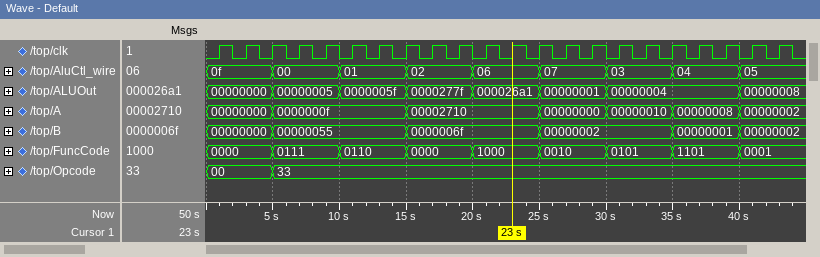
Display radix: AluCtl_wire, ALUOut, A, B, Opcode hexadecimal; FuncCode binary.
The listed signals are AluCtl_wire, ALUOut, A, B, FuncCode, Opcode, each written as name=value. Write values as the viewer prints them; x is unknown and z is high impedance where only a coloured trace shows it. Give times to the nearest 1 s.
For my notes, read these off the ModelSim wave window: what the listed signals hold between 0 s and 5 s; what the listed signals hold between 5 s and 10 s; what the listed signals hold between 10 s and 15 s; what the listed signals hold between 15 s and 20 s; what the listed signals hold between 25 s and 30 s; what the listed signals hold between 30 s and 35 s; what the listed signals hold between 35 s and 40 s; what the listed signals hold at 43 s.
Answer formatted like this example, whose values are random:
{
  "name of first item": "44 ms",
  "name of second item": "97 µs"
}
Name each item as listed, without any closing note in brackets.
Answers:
{
  "what the listed signals hold between 0 s and 5 s": "AluCtl_wire=0f, ALUOut=00000000, A=00000000, B=00000000, FuncCode=0000, Opcode=00",
  "what the listed signals hold between 5 s and 10 s": "AluCtl_wire=00, ALUOut=00000005, A=0000000f, B=00000055, FuncCode=0111, Opcode=33",
  "what the listed signals hold between 10 s and 15 s": "AluCtl_wire=01, ALUOut=0000005f, A=0000000f, B=00000055, FuncCode=0110, Opcode=33",
  "what the listed signals hold between 15 s and 20 s": "AluCtl_wire=02, ALUOut=0000277f, A=00002710, B=0000006f, FuncCode=0000, Opcode=33",
  "what the listed signals hold between 25 s and 30 s": "AluCtl_wire=07, ALUOut=00000001, A=00000000, B=00000002, FuncCode=0010, Opcode=33",
  "what the listed signals hold between 30 s and 35 s": "AluCtl_wire=03, ALUOut=00000004, A=00000010, B=00000002, FuncCode=0101, Opcode=33",
  "what the listed signals hold between 35 s and 40 s": "AluCtl_wire=04, ALUOut=00000004, A=00000008, B=00000001, FuncCode=1101, Opcode=33",
  "what the listed signals hold at 43 s": "AluCtl_wire=05, ALUOut=00000008, A=00000002, B=00000002, FuncCode=0001, Opcode=33"
}
